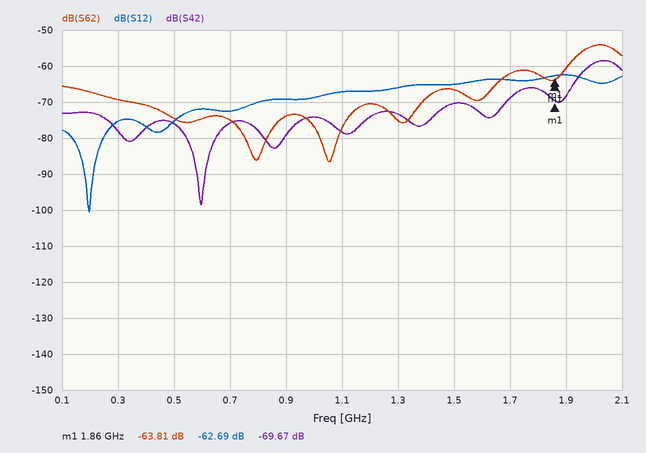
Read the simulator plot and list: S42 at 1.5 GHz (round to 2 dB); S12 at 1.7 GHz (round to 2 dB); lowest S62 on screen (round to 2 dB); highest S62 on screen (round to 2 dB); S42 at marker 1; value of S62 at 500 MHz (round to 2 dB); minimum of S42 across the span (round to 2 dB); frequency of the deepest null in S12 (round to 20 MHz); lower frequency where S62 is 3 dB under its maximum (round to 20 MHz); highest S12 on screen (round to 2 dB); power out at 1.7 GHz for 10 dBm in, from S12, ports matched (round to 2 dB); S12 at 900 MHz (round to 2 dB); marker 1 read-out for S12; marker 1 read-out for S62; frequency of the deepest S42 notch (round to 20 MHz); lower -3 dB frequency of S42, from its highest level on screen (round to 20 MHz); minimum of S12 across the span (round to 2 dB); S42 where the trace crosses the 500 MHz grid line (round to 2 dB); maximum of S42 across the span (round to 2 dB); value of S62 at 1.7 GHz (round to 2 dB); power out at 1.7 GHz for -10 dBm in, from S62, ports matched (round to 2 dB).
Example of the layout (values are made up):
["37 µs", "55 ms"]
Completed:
["-70 dB", "-64 dB", "-86 dB", "-54 dB", "-69.67 dB", "-74 dB", "-98 dB", "200 MHz", "1.94 GHz", "-62 dB", "-54 dBm", "-70 dB", "-62.69 dB", "-63.81 dB", "600 MHz", "1.96 GHz", "-100 dB", "-76 dB", "-58 dB", "-62 dB", "-72 dBm"]
